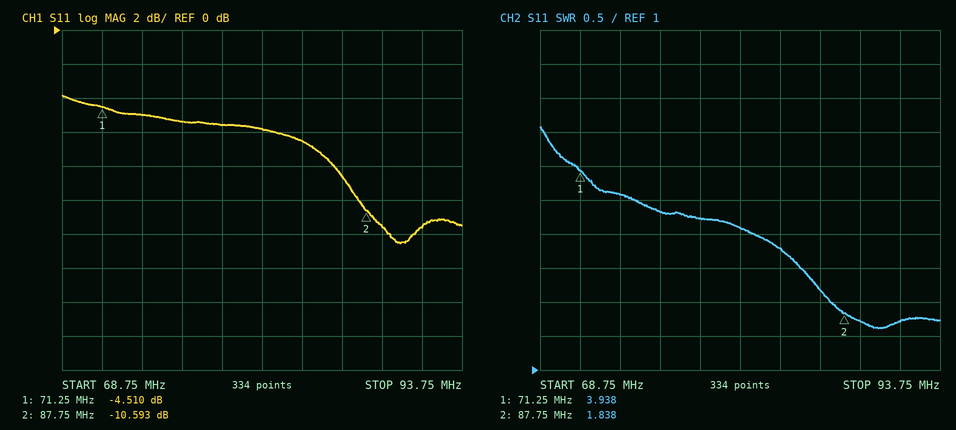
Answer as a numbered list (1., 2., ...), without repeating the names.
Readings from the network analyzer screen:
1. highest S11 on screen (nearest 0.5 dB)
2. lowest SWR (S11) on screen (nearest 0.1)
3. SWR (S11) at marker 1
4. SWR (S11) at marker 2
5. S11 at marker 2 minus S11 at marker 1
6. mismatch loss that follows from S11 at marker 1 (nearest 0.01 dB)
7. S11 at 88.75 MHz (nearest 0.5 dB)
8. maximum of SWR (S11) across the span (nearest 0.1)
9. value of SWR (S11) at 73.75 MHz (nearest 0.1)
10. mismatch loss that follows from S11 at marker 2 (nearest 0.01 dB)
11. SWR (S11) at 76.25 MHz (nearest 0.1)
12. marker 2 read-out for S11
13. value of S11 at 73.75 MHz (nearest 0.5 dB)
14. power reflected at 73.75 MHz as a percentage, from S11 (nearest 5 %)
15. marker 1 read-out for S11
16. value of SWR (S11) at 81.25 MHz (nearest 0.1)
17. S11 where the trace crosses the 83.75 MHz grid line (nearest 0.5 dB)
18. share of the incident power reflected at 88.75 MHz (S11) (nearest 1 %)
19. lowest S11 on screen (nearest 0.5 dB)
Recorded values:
1. -4.0 dB
2. 1.6
3. 3.938
4. 1.838
5. -6.083 dB
6. 1.90 dB
7. -11.5 dB
8. 4.6
9. 3.6
10. 0.40 dB
11. 3.3
12. -10.593 dB
13. -5.0 dB
14. 30 %
15. -4.510 dB
16. 3.1
17. -6.5 dB
18. 7 %
19. -12.5 dB
